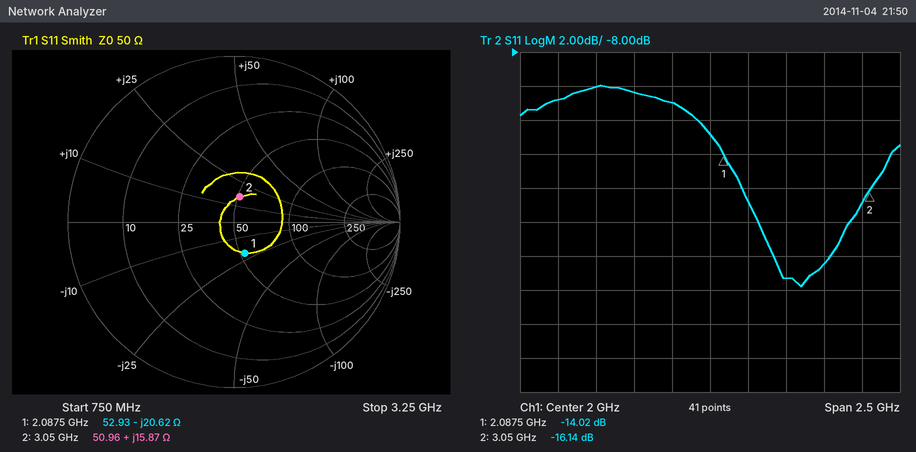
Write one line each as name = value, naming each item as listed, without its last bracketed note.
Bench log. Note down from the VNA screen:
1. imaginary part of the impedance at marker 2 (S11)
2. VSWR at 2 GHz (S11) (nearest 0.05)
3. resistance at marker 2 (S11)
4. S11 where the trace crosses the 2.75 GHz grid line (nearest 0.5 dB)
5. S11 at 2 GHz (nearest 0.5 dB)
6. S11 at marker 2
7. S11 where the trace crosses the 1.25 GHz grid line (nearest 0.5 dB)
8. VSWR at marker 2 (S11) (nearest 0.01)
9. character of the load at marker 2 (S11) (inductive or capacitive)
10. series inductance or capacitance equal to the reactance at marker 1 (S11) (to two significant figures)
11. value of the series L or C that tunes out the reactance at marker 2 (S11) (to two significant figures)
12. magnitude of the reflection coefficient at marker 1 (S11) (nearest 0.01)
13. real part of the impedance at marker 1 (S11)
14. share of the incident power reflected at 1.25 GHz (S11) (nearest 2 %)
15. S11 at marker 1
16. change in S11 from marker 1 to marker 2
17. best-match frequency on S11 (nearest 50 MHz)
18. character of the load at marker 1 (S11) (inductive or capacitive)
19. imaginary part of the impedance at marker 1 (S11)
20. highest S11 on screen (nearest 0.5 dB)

imaginary part of the impedance at marker 2 = +15.87 Ω
VSWR at 2 GHz (S11) = 1.60
resistance at marker 2 = 50.96 Ω
S11 where the trace crosses the 2.75 GHz grid line = -20.5 dB
S11 at 2 GHz = -13.0 dB
S11 at marker 2 = -16.14 dB
S11 where the trace crosses the 1.25 GHz grid line = -10.0 dB
VSWR at marker 2 (S11) = 1.37
character of the load at marker 2 (S11) = inductive
series inductance or capacitance equal to the reactance at marker 1 (S11) = 3.7 pF
value of the series L or C that tunes out the reactance at marker 2 (S11) = 3.3 pF
magnitude of the reflection coefficient at marker 1 (S11) = 0.20
real part of the impedance at marker 1 = 52.93 Ω
share of the incident power reflected at 1.25 GHz (S11) = 10 %
S11 at marker 1 = -14.02 dB
change in S11 from marker 1 to marker 2 = -2.12 dB
best-match frequency on S11 = 2.60 GHz
character of the load at marker 1 (S11) = capacitive
imaginary part of the impedance at marker 1 = -20.62 Ω
highest S11 on screen = -10.0 dB
